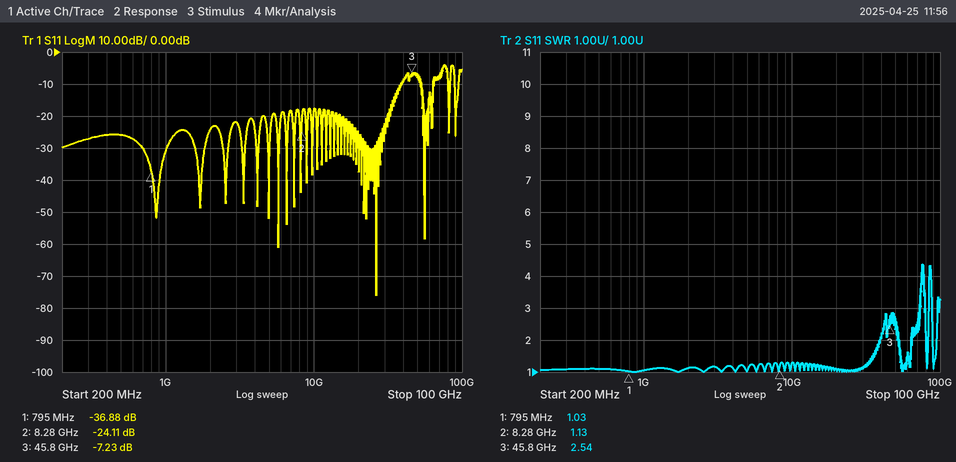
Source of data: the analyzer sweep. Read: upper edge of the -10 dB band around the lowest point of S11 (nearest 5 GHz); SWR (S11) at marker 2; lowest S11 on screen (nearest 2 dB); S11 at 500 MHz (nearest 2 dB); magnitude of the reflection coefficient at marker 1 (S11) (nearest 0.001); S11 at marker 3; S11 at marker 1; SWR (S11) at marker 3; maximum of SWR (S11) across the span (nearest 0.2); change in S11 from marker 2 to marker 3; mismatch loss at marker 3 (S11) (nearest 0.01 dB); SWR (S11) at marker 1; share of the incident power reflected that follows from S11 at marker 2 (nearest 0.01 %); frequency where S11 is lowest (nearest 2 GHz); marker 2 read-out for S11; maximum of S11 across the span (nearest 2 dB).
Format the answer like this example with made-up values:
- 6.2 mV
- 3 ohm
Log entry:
- 40 GHz
- 1.13
- -76 dB
- -26 dB
- 0.014
- -7.23 dB
- -36.88 dB
- 2.54
- 4.4
- 16.88 dB
- 0.91 dB
- 1.03
- 0.39 %
- 26 GHz
- -24.11 dB
- -4 dB
